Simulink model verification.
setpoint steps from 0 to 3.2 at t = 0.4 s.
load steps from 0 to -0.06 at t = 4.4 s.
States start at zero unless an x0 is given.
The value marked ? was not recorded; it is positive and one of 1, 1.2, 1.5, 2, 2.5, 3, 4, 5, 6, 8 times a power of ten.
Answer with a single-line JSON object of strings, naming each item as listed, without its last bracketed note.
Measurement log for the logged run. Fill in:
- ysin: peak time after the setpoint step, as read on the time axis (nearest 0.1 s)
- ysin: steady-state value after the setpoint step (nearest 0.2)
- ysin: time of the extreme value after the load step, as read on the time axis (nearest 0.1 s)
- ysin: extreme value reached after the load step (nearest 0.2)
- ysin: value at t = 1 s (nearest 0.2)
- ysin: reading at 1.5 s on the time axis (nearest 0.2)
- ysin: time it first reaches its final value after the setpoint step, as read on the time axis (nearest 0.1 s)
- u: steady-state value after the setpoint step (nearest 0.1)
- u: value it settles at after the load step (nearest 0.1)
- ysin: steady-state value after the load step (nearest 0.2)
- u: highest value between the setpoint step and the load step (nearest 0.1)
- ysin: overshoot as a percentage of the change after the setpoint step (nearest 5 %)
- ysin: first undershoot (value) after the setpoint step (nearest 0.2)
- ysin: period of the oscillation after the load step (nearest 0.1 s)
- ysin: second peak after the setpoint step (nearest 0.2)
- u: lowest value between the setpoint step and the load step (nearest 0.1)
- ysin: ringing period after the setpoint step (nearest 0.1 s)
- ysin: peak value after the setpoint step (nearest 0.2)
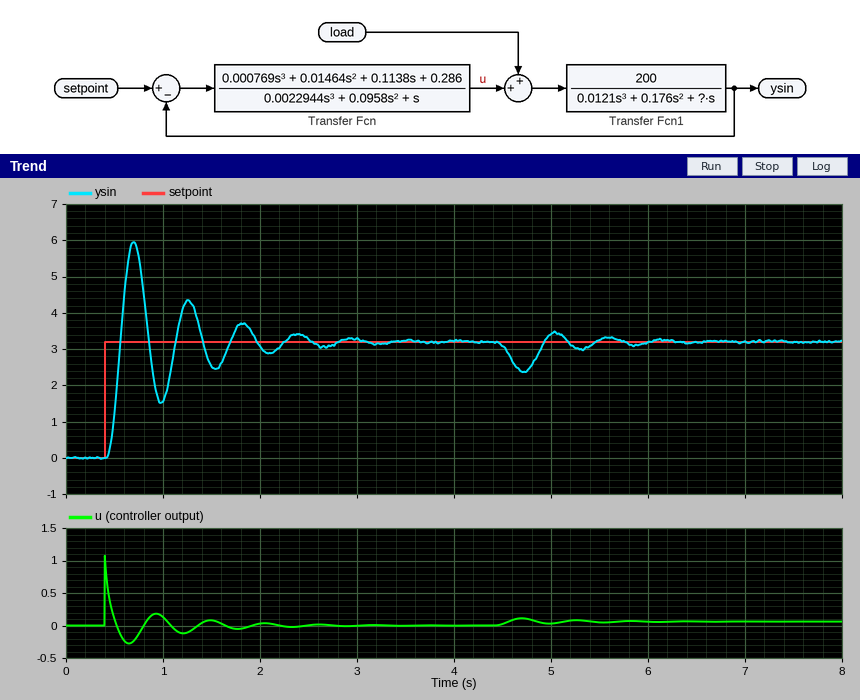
{"ysin: peak time after the setpoint step, as read on the time axis": "0.7 s", "ysin: steady-state value after the setpoint step": "3.2", "ysin: time of the extreme value after the load step, as read on the time axis": "4.7 s", "ysin: extreme value reached after the load step": "2.4", "ysin: value at t = 1 s": "1.6", "ysin: reading at 1.5 s on the time axis": "2.6", "ysin: time it first reaches its final value after the setpoint step, as read on the time axis": "0.6 s", "u: steady-state value after the setpoint step": "0.0", "u: value it settles at after the load step": "0.1", "ysin: steady-state value after the load step": "3.2", "u: highest value between the setpoint step and the load step": "1.1", "ysin: overshoot as a percentage of the change after the setpoint step": "85 %", "ysin: first undershoot (value) after the setpoint step": "1.6", "ysin: period of the oscillation after the load step": "0.6 s", "ysin: second peak after the setpoint step": "4.4", "u: lowest value between the setpoint step and the load step": "-0.3", "ysin: ringing period after the setpoint step": "0.6 s", "ysin: peak value after the setpoint step": "6.0"}
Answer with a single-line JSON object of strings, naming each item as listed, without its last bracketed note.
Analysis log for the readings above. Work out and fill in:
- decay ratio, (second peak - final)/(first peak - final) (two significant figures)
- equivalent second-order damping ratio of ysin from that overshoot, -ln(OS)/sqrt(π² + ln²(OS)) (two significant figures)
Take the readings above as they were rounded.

{"decay ratio, (second peak - final)/(first peak - final)": "0.43", "equivalent second-order damping ratio of ysin from that overshoot, -ln(OS)/sqrt(π² + ln²(OS))": "0.052"}
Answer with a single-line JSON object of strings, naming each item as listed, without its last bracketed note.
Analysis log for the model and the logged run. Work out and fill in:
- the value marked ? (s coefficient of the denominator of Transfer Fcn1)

{"the value marked ?": "1"}
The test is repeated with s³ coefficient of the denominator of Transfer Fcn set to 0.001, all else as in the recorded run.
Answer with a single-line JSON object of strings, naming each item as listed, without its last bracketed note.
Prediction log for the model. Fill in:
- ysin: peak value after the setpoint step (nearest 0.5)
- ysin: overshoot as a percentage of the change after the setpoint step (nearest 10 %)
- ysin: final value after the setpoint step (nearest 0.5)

{"ysin: peak value after the setpoint step": "5.5", "ysin: overshoot as a percentage of the change after the setpoint step": "70 %", "ysin: final value after the setpoint step": "3.0"}
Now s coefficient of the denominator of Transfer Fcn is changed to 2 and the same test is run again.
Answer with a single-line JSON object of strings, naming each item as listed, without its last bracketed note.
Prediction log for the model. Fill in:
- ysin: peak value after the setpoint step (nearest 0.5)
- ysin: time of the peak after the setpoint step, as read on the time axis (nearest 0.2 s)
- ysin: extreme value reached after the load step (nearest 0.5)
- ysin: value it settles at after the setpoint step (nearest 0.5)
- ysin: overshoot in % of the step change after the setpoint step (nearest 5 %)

{"ysin: peak value after the setpoint step": "4.5", "ysin: time of the peak after the setpoint step, as read on the time axis": "0.8 s", "ysin: extreme value reached after the load step": "2.0", "ysin: value it settles at after the setpoint step": "3.0", "ysin: overshoot in % of the step change after the setpoint step": "40 %"}
